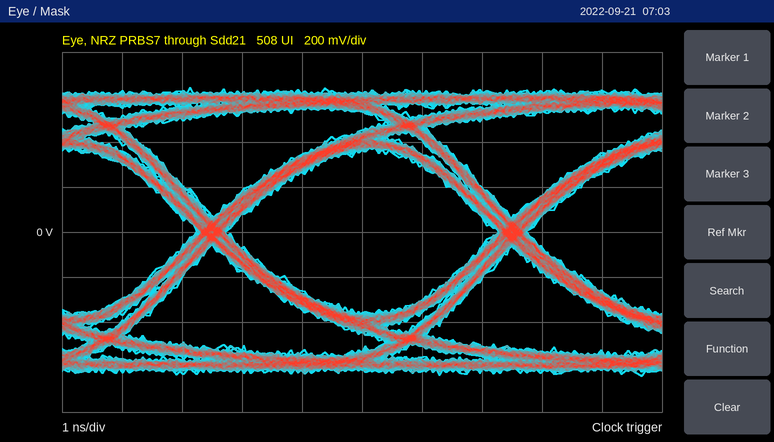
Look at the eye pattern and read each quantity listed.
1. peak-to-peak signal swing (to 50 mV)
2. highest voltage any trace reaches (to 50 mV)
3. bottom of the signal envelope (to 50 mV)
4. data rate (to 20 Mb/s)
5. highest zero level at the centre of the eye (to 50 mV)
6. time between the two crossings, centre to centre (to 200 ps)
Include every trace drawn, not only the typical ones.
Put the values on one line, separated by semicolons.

1.30 V; 650 mV; -650 mV; 200 Mb/s; -350 mV; 5.0 ns
